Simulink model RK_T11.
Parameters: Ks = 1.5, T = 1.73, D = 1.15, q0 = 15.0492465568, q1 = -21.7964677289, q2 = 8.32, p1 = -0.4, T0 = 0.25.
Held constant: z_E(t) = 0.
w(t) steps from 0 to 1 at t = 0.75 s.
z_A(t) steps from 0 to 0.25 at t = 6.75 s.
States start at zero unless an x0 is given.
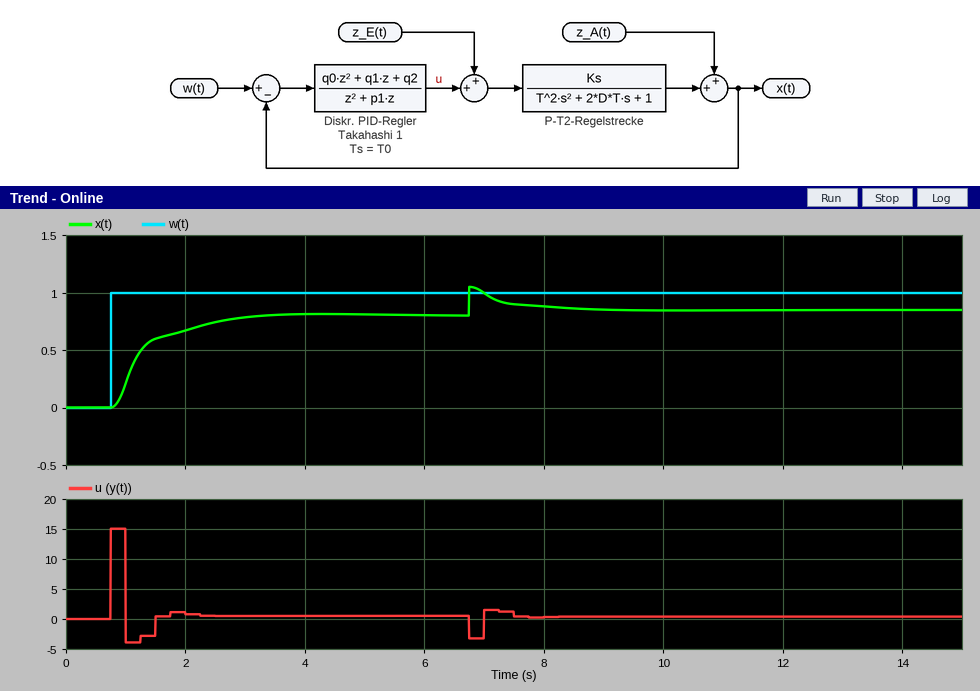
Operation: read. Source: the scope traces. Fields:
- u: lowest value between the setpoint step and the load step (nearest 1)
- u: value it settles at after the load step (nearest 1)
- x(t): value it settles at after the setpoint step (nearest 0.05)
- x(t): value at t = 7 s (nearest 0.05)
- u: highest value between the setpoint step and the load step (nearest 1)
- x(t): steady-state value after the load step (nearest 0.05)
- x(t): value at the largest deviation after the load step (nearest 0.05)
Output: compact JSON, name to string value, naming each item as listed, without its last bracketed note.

{"u: lowest value between the setpoint step and the load step": "-4", "u: value it settles at after the load step": "0", "x(t): value it settles at after the setpoint step": "0.80", "x(t): value at t = 7 s": "1.00", "u: highest value between the setpoint step and the load step": "15", "x(t): steady-state value after the load step": "0.85", "x(t): value at the largest deviation after the load step": "1.05"}
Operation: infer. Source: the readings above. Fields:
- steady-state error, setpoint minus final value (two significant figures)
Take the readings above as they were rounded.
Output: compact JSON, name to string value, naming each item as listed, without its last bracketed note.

{"steady-state error, setpoint minus final value": "0.20"}
